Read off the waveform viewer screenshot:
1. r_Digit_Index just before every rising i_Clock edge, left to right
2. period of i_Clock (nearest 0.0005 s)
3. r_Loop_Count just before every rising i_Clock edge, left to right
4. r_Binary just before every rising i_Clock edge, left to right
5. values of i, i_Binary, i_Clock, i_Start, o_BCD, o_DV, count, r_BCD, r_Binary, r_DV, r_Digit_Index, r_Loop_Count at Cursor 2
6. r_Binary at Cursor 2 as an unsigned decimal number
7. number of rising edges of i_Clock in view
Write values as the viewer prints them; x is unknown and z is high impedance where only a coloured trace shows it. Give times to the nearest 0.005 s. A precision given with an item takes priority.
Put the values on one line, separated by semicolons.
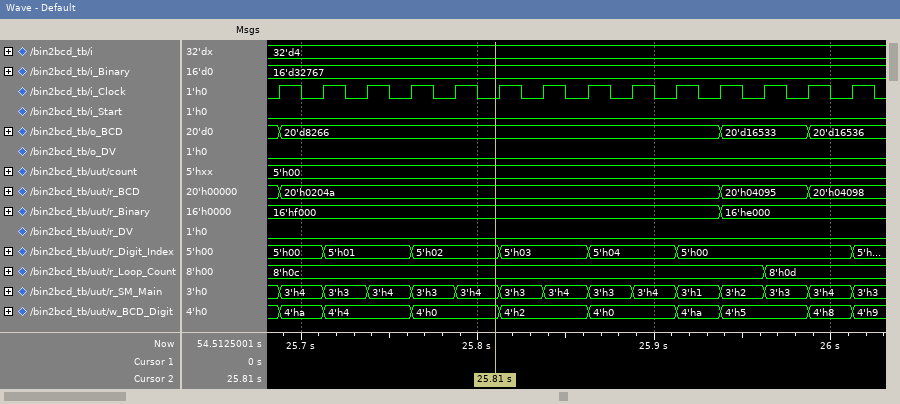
5'h00, 5'h00, 5'h01, 5'h01, 5'h02, 5'h02, 5'h03, 5'h03, 5'h04, 5'h04, 5'h00, 5'h00, 5'h00, 5'h00; 0.025 s; 8'h0c, 8'h0c, 8'h0c, 8'h0c, 8'h0c, 8'h0c, 8'h0c, 8'h0c, 8'h0c, 8'h0c, 8'h0c, 8'h0c, 8'h0d, 8'h0d; 16'hf000, 16'hf000, 16'hf000, 16'hf000, 16'hf000, 16'hf000, 16'hf000, 16'hf000, 16'hf000, 16'hf000, 16'hf000, 16'he000, 16'he000, 16'he000; i=32'd4, i_Binary=16'd32767, i_Clock=0, i_Start=0, o_BCD=20'd8266, o_DV=0, count=5'h00, r_BCD=20'h0204a, r_Binary=16'hf000, r_DV=0, r_Digit_Index=5'h02, r_Loop_Count=8'h0c; 61440; 14
